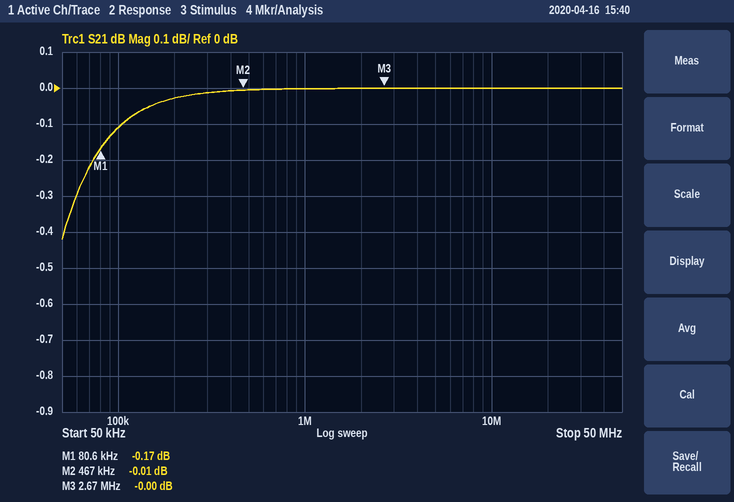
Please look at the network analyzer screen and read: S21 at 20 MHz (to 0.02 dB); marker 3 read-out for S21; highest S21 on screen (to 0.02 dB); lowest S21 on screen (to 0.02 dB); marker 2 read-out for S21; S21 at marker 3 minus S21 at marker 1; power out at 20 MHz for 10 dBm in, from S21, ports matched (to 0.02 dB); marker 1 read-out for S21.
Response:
0.00 dB
-0.00 dB
0.00 dB
-0.42 dB
-0.01 dB
0.17 dB
10.00 dBm
-0.17 dB
